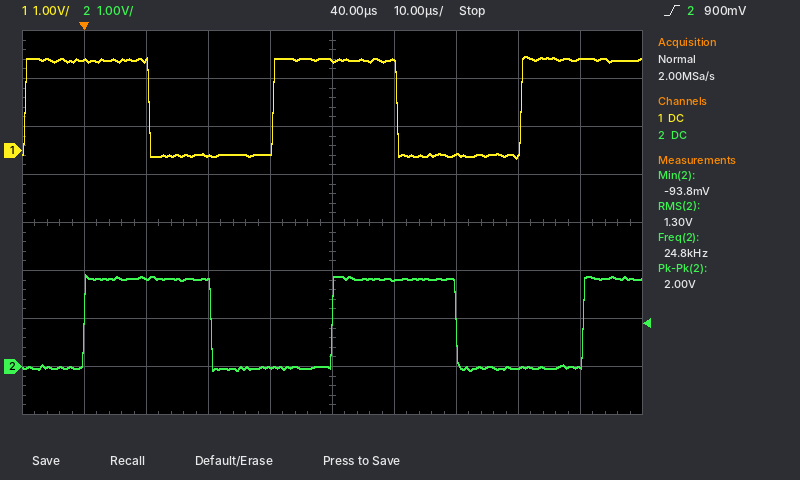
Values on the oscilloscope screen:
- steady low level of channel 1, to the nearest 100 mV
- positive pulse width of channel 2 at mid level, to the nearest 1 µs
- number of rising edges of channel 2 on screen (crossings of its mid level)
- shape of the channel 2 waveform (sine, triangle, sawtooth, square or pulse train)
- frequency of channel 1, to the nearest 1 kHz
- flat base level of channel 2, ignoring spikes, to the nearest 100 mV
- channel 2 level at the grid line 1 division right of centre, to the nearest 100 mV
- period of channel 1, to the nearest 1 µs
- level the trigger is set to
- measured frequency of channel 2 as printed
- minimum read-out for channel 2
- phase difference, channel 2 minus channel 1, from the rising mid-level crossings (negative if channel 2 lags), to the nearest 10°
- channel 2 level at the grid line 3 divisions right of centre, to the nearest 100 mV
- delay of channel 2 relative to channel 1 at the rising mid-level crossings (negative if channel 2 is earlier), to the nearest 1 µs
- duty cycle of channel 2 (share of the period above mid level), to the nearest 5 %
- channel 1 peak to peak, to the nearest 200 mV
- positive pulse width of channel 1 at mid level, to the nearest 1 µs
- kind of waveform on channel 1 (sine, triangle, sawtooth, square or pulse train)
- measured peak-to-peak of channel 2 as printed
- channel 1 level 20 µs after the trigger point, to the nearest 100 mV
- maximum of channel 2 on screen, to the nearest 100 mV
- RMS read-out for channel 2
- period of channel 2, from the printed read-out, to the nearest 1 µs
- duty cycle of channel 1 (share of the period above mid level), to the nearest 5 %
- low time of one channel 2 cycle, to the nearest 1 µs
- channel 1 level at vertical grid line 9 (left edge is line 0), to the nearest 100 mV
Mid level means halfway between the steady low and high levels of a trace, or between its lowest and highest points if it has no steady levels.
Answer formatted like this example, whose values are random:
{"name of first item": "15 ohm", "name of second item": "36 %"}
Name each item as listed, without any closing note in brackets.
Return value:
{"steady low level of channel 1, to the nearest 100 mV": "-100 mV", "positive pulse width of channel 2 at mid level, to the nearest 1 µs": "20 µs", "number of rising edges of channel 2 on screen": "3", "shape of the channel 2 waveform": "square", "frequency of channel 1, to the nearest 1 kHz": "25 kHz", "flat base level of channel 2, ignoring spikes, to the nearest 100 mV": "0.0 V", "channel 2 level at the grid line 1 division right of centre, to the nearest 100 mV": "1.8 V", "period of channel 1, to the nearest 1 µs": "40 µs", "level the trigger is set to": "900 mV", "measured frequency of channel 2 as printed": "24.8 kHz", "minimum read-out for channel 2": "-93.8 mV", "phase difference, channel 2 minus channel 1, from the rising mid-level crossings (negative if channel 2 lags), to the nearest 10°": "-90°", "channel 2 level at the grid line 3 divisions right of centre, to the nearest 100 mV": "0.0 V", "delay of channel 2 relative to channel 1 at the rising mid-level crossings (negative if channel 2 is earlier), to the nearest 1 µs": "+10 µs", "duty cycle of channel 2 (share of the period above mid level), to the nearest 5 %": "50 %", "channel 1 peak to peak, to the nearest 200 mV": "2.2 V", "positive pulse width of channel 1 at mid level, to the nearest 1 µs": "20 µs", "kind of waveform on channel 1": "square", "measured peak-to-peak of channel 2 as printed": "2.00 V", "channel 1 level 20 µs after the trigger point, to the nearest 100 mV": "-100 mV", "maximum of channel 2 on screen, to the nearest 100 mV": "1.9 V", "RMS read-out for channel 2": "1.30 V", "period of channel 2, from the printed read-out, to the nearest 1 µs": "40 µs", "duty cycle of channel 1 (share of the period above mid level), to the nearest 5 %": "50 %", "low time of one channel 2 cycle, to the nearest 1 µs": "20 µs", "channel 1 level at vertical grid line 9 (left edge is line 0), to the nearest 100 mV": "1.9 V"}
